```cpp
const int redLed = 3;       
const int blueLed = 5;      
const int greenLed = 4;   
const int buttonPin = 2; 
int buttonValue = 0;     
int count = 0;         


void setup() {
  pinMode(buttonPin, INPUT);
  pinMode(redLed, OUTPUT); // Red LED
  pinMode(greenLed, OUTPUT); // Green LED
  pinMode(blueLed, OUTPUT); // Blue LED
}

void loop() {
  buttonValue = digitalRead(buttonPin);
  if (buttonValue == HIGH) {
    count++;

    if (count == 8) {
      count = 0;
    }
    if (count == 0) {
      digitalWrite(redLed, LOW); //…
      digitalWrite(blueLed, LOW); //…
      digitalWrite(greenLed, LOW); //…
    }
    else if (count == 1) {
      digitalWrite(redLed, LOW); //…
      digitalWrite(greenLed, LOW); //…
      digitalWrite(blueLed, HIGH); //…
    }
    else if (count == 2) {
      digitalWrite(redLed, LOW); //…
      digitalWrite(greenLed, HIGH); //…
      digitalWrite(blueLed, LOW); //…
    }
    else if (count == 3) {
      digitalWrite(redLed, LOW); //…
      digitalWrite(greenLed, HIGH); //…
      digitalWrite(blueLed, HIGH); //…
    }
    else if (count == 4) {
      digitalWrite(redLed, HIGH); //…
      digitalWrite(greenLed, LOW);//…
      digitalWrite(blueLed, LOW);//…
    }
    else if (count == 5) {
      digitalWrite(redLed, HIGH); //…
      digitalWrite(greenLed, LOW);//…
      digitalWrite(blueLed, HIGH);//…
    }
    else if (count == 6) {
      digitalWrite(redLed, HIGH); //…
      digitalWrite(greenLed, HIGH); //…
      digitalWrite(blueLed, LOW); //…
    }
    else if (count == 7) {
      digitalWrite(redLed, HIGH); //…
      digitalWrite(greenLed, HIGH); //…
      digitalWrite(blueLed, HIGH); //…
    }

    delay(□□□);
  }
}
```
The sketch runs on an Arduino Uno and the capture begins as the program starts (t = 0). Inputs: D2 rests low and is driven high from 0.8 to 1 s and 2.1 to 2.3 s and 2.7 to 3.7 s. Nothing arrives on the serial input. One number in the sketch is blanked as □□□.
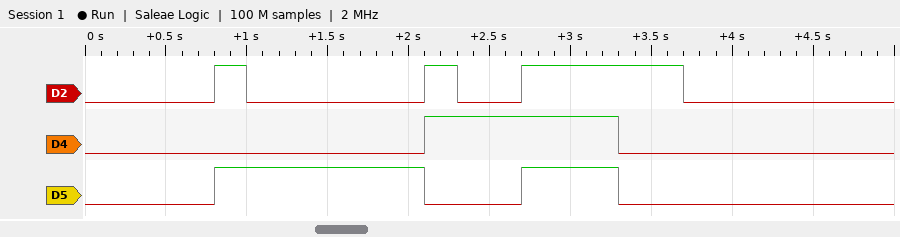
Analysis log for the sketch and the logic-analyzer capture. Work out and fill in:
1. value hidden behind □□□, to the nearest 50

600
